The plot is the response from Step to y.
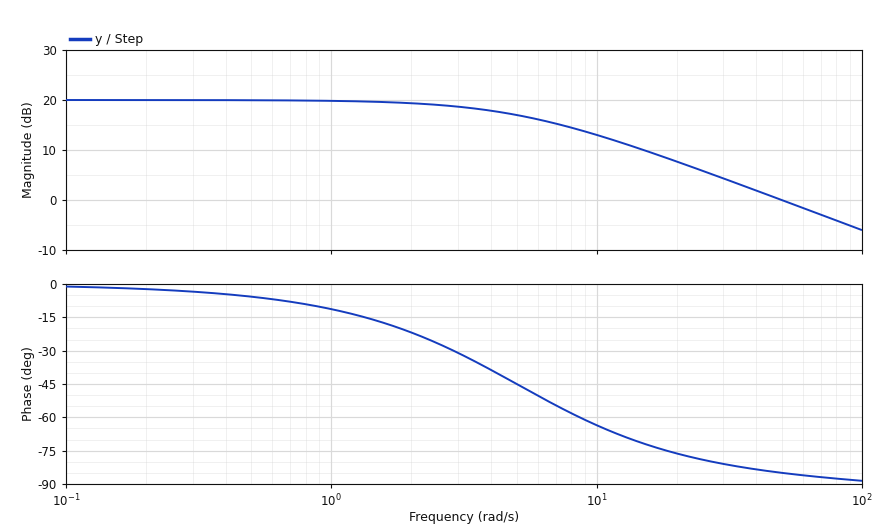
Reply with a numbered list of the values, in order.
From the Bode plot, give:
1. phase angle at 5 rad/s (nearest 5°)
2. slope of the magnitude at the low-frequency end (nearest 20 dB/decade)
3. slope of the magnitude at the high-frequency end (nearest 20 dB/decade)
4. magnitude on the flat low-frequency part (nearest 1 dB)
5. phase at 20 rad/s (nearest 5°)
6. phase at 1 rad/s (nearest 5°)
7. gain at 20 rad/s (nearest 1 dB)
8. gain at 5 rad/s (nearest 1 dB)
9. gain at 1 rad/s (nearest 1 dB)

1. -45°
2. 0 dB/decade
3. -20 dB/decade
4. 20 dB
5. -75°
6. -10°
7. 8 dB
8. 17 dB
9. 20 dB
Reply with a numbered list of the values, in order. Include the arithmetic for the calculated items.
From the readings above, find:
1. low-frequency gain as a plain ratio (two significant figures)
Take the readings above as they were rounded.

1. 10^(20 / 20) = 10
